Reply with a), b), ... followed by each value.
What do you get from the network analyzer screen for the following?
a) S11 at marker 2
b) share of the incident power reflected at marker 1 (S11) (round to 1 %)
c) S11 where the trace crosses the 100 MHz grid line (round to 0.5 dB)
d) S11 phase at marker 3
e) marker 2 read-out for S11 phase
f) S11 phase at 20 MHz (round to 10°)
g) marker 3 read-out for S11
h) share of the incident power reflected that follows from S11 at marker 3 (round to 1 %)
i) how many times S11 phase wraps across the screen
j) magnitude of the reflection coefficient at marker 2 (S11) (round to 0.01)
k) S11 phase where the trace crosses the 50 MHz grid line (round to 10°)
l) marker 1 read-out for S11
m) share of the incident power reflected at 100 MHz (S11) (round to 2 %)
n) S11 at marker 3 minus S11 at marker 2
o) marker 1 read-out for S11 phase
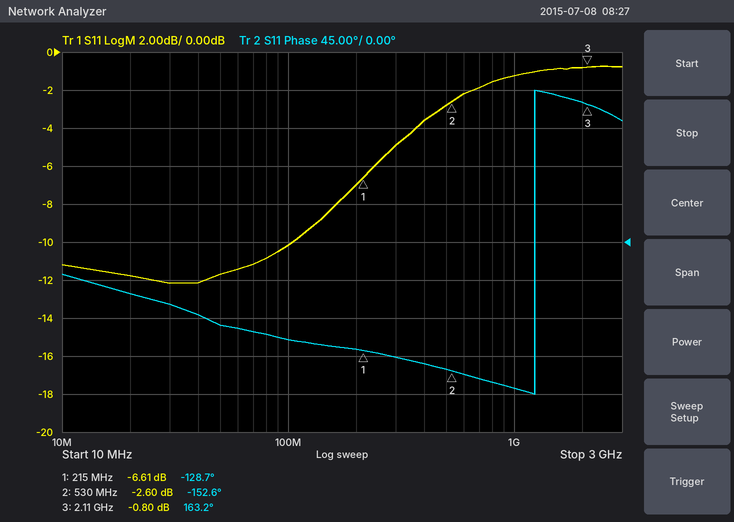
a) -2.60 dB
b) 22 %
c) -10.0 dB
d) 163.2°
e) -152.6°
f) -60°
g) -0.80 dB
h) 83 %
i) 1
j) 0.74
k) -100°
l) -6.61 dB
m) 10 %
n) 1.80 dB
o) -128.7°
